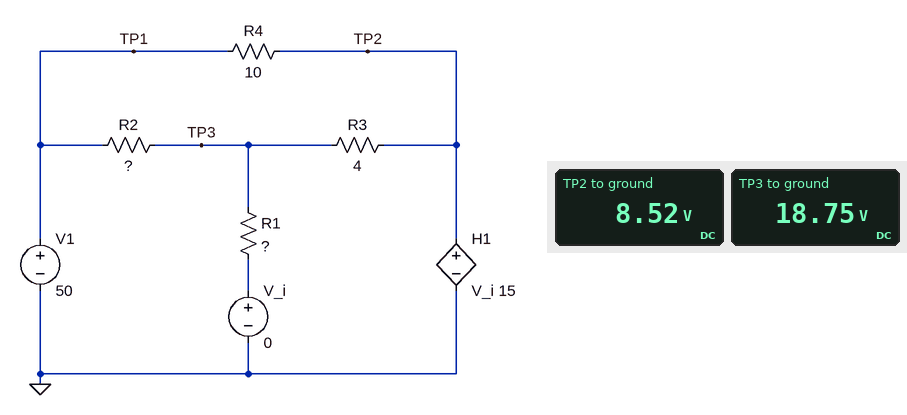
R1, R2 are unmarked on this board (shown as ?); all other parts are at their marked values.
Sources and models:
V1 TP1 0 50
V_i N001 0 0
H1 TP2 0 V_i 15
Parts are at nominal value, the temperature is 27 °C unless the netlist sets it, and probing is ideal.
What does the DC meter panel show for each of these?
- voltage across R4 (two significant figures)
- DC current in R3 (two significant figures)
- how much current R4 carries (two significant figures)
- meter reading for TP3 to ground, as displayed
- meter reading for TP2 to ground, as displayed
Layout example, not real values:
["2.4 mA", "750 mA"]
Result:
["41 V", "2.6 A", "4.1 A", "18.75 V", "8.52 V"]
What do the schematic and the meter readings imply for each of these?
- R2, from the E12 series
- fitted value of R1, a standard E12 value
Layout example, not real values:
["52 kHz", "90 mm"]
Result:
["10 Ω", "33 Ω"]
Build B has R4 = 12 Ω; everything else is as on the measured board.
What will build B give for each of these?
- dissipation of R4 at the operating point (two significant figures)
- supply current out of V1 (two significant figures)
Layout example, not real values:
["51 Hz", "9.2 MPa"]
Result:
["140 W", "6.6 A"]
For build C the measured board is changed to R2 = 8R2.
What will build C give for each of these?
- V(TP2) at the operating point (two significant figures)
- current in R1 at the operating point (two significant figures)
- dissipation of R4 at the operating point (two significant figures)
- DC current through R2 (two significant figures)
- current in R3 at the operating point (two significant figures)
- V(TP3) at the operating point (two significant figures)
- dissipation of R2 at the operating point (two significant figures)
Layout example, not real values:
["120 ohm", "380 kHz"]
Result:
["9.6 V", "640 mA", "160 W", "3.5 A", "2.9 A", "21 V", "100 W"]
